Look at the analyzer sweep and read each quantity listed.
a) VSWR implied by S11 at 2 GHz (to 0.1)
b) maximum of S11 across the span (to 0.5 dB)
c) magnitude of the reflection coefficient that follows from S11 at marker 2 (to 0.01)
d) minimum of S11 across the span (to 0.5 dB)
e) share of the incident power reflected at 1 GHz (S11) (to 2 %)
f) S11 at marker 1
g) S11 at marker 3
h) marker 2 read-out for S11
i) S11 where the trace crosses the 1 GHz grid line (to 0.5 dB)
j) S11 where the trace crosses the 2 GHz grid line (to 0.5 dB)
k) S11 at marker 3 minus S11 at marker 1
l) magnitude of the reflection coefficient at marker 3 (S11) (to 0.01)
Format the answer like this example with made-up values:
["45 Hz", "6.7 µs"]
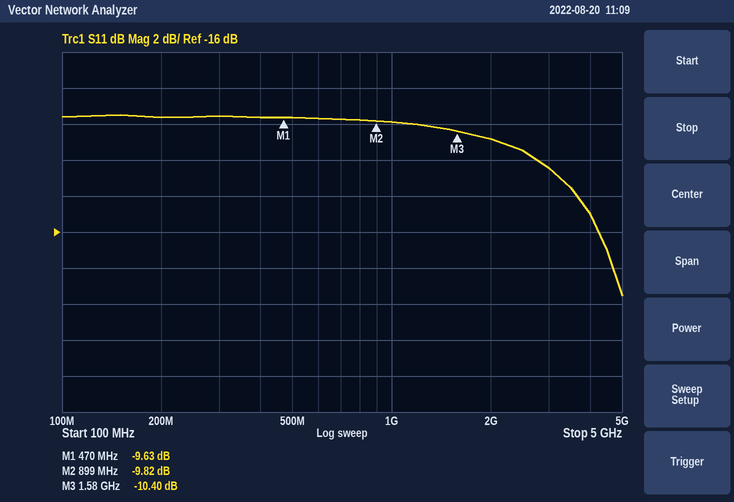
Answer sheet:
["1.8", "-9.5 dB", "0.32", "-19.5 dB", "10 %", "-9.63 dB", "-10.40 dB", "-9.82 dB", "-10.0 dB", "-11.0 dB", "-0.77 dB", "0.30"]
